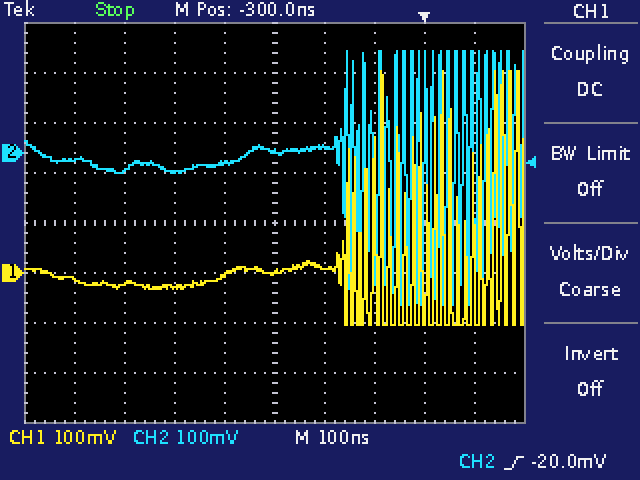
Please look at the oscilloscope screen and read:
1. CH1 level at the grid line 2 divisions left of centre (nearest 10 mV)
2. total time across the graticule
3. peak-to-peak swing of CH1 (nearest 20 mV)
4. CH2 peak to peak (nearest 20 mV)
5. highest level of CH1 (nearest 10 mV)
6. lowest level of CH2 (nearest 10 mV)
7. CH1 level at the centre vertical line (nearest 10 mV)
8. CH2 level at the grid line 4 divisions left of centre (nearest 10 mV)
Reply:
-30 mV
1 µs
500 mV
500 mV
400 mV
-300 mV
0 mV
-10 mV
